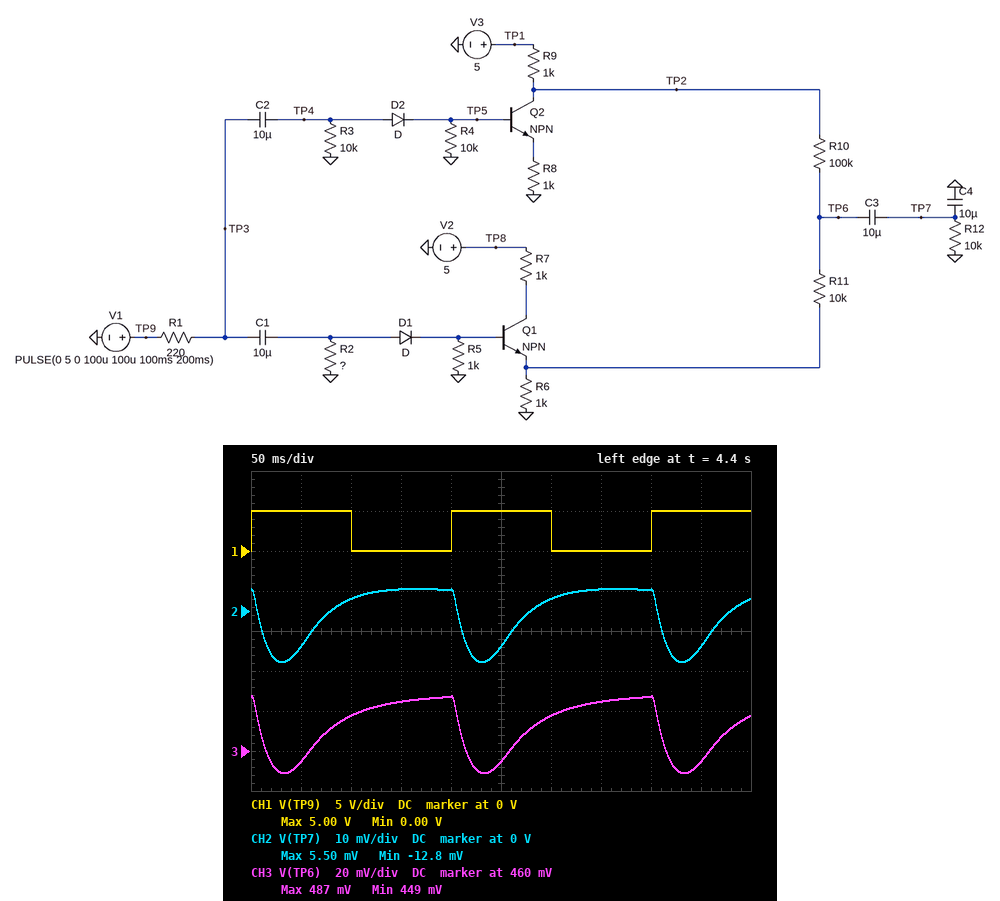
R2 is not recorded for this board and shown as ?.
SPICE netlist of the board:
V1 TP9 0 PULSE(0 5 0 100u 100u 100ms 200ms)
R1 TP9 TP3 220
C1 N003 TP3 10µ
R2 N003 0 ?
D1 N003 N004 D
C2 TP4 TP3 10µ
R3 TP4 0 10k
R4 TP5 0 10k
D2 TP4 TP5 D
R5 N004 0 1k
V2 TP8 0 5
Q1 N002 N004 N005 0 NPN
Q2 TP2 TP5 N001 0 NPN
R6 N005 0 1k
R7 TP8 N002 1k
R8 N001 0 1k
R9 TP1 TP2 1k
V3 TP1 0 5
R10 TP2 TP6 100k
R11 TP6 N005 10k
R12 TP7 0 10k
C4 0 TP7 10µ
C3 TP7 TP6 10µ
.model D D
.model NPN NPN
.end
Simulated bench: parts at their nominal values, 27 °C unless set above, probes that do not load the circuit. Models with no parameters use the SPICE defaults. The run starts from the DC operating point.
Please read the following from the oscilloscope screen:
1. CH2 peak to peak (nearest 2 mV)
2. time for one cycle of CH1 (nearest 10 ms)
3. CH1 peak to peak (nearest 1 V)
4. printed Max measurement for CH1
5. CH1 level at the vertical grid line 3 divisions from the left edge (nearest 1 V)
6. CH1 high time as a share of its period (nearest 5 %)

18 mV
200 ms
5 V
5.00 V
0 V
50 %
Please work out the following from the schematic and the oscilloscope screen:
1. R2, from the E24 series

24 kΩ
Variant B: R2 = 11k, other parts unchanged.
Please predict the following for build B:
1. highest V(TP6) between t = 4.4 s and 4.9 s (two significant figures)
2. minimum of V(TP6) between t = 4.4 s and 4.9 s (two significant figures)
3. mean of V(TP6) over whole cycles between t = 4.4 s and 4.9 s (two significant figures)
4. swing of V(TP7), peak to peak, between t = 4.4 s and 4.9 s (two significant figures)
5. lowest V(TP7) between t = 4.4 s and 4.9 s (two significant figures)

540 mV
480 mV
490 mV
31 mV
-5.9 mV
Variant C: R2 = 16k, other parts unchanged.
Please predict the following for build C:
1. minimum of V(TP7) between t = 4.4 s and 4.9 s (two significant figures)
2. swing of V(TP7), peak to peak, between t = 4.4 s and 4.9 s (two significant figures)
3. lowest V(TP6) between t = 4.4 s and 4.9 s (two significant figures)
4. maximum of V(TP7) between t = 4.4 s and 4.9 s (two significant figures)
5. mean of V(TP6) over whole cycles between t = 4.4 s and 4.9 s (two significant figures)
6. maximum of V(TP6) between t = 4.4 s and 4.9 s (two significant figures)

-9.1 mV
21 mV
460 mV
12 mV
480 mV
510 mV
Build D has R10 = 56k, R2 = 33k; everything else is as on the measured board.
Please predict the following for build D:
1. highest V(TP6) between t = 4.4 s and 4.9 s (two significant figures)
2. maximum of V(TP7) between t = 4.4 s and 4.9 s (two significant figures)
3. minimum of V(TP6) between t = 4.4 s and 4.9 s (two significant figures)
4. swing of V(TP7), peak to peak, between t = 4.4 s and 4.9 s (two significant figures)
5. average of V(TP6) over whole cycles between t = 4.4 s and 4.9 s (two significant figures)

800 mV
10 mV
730 mV
35 mV
780 mV
